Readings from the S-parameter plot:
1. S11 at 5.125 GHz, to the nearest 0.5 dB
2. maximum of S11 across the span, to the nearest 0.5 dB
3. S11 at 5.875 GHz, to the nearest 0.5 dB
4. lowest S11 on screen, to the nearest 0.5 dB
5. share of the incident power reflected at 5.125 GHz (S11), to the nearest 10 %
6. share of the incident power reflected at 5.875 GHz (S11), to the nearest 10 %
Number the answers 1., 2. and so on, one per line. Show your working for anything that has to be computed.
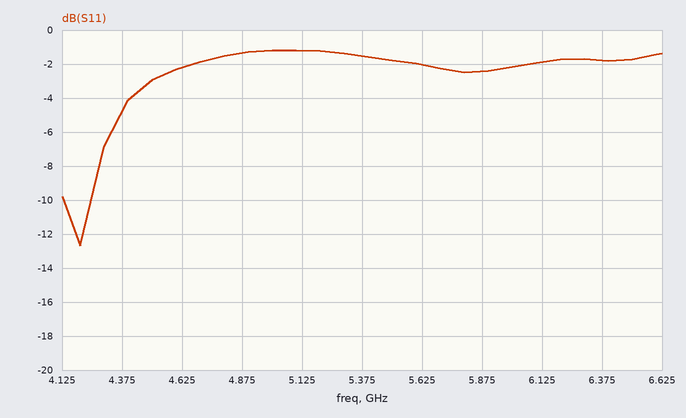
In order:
1. -1.0 dB
2. -1.0 dB
3. -2.5 dB
4. -12.5 dB
5. 10^(-1/10) ≈ 79.4 %, so 80 % to the nearest 10 %
6. 10^(-2.5/10) ≈ 56.2 %, so 60 % to the nearest 10 %
